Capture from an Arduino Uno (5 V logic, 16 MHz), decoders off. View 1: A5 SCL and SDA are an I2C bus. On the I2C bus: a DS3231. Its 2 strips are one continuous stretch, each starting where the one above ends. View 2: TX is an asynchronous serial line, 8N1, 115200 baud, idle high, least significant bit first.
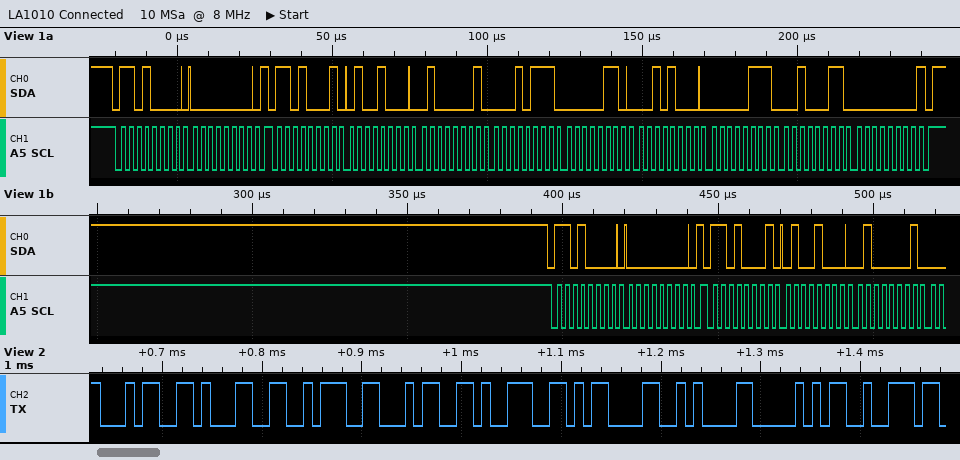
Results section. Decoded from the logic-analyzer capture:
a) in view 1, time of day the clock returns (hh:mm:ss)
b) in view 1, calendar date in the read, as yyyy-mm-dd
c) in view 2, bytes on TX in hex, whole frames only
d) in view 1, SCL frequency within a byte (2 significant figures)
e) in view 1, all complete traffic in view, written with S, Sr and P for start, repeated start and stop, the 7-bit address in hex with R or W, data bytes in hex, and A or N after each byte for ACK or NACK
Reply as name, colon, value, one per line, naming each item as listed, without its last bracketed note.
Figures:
in view 1, time of day the clock returns: 17:41:48
in view 1, calendar date in the read, as yyyy-mm-dd: 2023-07-28
in view 2, bytes on TX in hex, whole frames only: 34 31 3A 34 39 0D 0A 50 72
in view 1, SCL frequency within a byte: 400 kHz
in view 1, all complete traffic in view, written with S, Sr and P for start, repeated start and stop, the 7-bit address in hex with R or W, data bytes in hex, and A or N after each byte for ACK or NACK: S 68W A 00 A Sr 68R A 48 A 41 A 17 A 06 A 28 A 07 A 23 A 00 N P S 68W A 00 A Sr 68R A 48 A 41 A
